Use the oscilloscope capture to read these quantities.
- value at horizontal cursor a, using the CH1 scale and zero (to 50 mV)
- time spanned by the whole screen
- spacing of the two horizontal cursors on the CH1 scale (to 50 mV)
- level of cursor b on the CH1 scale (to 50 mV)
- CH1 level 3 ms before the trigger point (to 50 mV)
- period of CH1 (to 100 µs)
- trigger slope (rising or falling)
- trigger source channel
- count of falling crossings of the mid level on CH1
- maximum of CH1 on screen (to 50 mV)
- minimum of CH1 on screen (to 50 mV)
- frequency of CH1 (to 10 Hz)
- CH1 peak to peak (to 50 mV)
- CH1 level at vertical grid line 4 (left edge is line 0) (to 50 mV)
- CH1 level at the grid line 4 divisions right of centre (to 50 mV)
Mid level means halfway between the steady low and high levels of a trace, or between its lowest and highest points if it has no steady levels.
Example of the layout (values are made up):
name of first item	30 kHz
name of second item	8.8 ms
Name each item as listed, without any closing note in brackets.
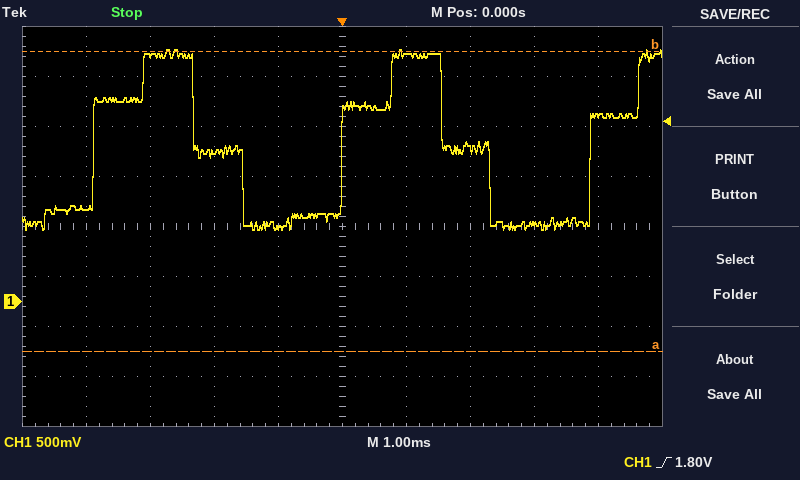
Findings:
value at horizontal cursor a, using the CH1 scale and zero	-500 mV
time spanned by the whole screen	10 ms
spacing of the two horizontal cursors on the CH1 scale	3.00 V
level of cursor b on the CH1 scale	2.50 V
CH1 level 3 ms before the trigger point	2.45 V
period of CH1	3.9 ms
trigger slope	rising
trigger source channel	CH1
count of falling crossings of the mid level on CH1	2
maximum of CH1 on screen	2.50 V
minimum of CH1 on screen	700 mV
frequency of CH1	260 Hz
CH1 peak to peak	1.80 V
CH1 level at vertical grid line 4 (left edge is line 0)	750 mV
CH1 level at the grid line 4 divisions right of centre	1.85 V
